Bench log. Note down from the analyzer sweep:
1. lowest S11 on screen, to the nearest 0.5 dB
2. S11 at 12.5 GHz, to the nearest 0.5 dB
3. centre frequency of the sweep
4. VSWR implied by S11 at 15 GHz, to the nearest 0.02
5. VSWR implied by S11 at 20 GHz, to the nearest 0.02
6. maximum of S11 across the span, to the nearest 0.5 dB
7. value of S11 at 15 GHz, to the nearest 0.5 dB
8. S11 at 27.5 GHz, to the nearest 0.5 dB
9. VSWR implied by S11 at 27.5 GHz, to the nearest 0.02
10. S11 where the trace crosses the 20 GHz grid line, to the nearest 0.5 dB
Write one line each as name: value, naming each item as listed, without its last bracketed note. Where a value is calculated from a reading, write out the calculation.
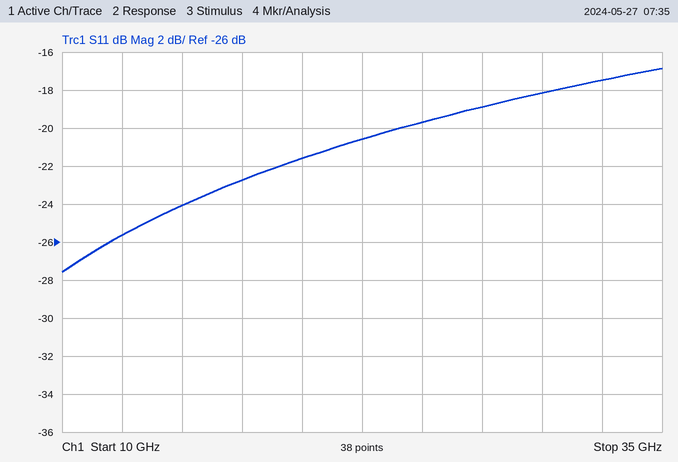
lowest S11 on screen, to the nearest 0.5 dB: -27.5 dB
S11 at 12.5 GHz, to the nearest 0.5 dB: -25.5 dB
centre frequency of the sweep: 22.5 GHz
VSWR implied by S11 at 15 GHz, to the nearest 0.02: |Γ| = 10^(-24/20) = 0.0631; VSWR = (1 + 0.0631)/(1 − 0.0631) ≈ 1.13, so 1.14 to the nearest 0.02
VSWR implied by S11 at 20 GHz, to the nearest 0.02: |Γ| = 10^(-21.5/20) = 0.0841; VSWR = (1 + 0.0841)/(1 − 0.0841) ≈ 1.18
maximum of S11 across the span, to the nearest 0.5 dB: -17.0 dB
value of S11 at 15 GHz, to the nearest 0.5 dB: -24.0 dB
S11 at 27.5 GHz, to the nearest 0.5 dB: -19.0 dB
VSWR implied by S11 at 27.5 GHz, to the nearest 0.02: |Γ| = 10^(-19/20) = 0.1122; VSWR = (1 + 0.1122)/(1 − 0.1122) ≈ 1.25, so 1.26 to the nearest 0.02
S11 where the trace crosses the 20 GHz grid line, to the nearest 0.5 dB: -21.5 dB
